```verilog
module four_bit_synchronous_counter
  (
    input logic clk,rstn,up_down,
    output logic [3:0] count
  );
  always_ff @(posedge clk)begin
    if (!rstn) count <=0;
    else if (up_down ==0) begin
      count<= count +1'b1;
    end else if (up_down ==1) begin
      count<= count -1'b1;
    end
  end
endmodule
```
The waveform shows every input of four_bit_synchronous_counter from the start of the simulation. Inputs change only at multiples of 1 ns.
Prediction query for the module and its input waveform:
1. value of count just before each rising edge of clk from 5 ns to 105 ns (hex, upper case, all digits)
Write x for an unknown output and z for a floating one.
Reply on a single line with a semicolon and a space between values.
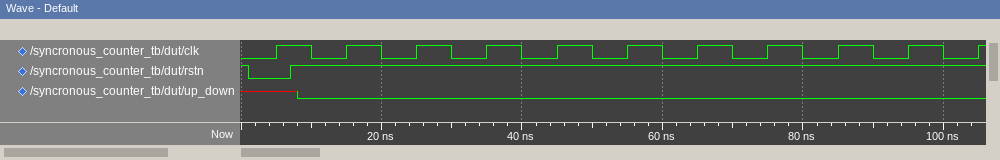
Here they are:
x, 0, 1, 2, 3, 4, 5, 6, 7, 8, 9
